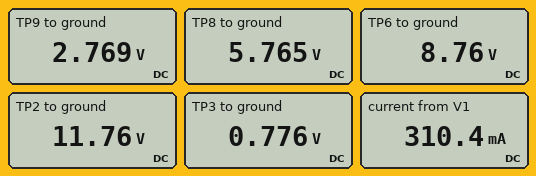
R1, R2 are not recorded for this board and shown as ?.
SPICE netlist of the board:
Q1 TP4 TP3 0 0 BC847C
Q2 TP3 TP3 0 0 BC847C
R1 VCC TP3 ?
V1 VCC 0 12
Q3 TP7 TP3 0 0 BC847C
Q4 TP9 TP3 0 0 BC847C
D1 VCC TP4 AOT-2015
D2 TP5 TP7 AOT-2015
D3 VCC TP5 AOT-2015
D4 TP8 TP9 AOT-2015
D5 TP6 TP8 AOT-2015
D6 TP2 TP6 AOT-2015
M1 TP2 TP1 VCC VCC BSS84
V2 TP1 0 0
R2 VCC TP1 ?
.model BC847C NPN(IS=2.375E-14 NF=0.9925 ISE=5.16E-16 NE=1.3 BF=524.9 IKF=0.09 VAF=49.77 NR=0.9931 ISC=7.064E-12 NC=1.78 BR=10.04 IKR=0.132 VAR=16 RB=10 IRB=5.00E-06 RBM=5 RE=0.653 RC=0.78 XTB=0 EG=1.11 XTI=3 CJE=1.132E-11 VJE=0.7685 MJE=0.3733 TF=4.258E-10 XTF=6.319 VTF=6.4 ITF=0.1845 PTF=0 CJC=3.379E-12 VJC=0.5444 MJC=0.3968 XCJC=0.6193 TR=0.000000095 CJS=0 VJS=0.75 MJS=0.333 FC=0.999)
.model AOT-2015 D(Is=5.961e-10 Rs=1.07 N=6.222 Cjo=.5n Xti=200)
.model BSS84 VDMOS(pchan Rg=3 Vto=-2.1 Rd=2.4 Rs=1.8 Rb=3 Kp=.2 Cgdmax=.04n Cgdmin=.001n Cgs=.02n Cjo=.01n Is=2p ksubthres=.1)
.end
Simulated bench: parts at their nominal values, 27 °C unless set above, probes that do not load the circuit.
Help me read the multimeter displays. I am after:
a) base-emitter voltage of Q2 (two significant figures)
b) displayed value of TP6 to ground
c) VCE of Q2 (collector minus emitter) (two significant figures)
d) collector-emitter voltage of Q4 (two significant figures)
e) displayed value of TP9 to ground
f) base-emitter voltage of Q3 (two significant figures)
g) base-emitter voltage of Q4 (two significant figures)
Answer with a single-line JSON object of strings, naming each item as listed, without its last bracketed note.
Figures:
{"base-emitter voltage of Q2": "780 mV", "displayed value of TP6 to ground": "8.76 V", "VCE of Q2 (collector minus emitter)": "780 mV", "collector-emitter voltage of Q4": "2.8 V", "displayed value of TP9 to ground": "2.769 V", "base-emitter voltage of Q3": "780 mV", "base-emitter voltage of Q4": "780 mV"}
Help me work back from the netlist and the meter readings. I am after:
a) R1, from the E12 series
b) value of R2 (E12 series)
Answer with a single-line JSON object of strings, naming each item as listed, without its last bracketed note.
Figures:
{"R1, from the E12 series": "220 Ω", "value of R2": "120 Ω"}
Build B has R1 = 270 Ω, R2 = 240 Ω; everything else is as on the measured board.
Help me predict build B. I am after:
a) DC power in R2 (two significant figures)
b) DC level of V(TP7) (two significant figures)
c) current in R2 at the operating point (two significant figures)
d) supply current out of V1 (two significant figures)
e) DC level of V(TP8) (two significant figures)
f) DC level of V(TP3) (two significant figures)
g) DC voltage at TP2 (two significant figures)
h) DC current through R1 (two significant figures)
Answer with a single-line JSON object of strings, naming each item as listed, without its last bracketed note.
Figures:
{"DC power in R2": "600 mW", "DC level of V(TP7)": "6.1 V", "current in R2 at the operating point": "50 mA", "supply current out of V1": "220 mA", "DC level of V(TP8)": "5.9 V", "DC level of V(TP3)": "760 mV", "DC voltage at TP2": "12 V", "DC current through R1": "42 mA"}
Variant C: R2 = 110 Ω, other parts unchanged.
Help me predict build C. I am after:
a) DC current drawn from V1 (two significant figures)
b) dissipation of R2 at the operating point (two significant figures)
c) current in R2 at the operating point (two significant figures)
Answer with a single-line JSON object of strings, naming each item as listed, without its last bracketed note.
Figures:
{"DC current drawn from V1": "320 mA", "dissipation of R2 at the operating point": "1.3 W", "current in R2 at the operating point": "110 mA"}
